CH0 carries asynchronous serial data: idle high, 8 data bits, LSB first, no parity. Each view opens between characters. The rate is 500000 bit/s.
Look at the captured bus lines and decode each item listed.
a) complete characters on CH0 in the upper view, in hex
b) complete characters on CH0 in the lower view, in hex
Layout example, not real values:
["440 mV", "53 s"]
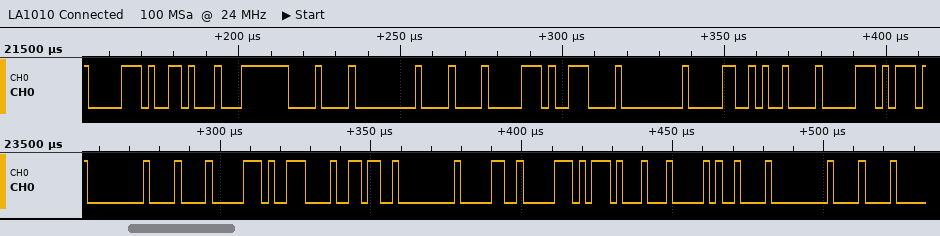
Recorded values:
["70, 16, FC, 08, 00, 08, 70, 0E, 00, 30, 09, 70", "00, 08, 70, 0E, 36, 00, 30, 70, 17, 04, 09, 00, 08"]
